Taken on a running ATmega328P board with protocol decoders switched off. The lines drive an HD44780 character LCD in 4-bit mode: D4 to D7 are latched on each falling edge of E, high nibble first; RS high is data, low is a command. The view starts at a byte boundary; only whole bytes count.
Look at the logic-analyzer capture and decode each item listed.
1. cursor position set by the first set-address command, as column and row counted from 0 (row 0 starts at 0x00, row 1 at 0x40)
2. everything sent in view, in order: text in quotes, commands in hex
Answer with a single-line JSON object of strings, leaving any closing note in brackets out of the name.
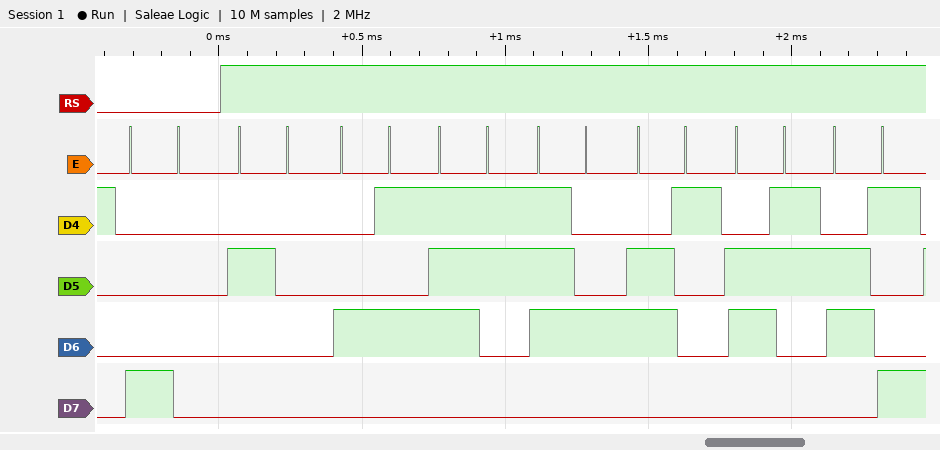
{"cursor position set by the first set-address command, as column and row counted from 0": "column 0, row 0", "everything sent in view, in order: text in quotes, commands in hex": "0x80 \" Estaci\""}
